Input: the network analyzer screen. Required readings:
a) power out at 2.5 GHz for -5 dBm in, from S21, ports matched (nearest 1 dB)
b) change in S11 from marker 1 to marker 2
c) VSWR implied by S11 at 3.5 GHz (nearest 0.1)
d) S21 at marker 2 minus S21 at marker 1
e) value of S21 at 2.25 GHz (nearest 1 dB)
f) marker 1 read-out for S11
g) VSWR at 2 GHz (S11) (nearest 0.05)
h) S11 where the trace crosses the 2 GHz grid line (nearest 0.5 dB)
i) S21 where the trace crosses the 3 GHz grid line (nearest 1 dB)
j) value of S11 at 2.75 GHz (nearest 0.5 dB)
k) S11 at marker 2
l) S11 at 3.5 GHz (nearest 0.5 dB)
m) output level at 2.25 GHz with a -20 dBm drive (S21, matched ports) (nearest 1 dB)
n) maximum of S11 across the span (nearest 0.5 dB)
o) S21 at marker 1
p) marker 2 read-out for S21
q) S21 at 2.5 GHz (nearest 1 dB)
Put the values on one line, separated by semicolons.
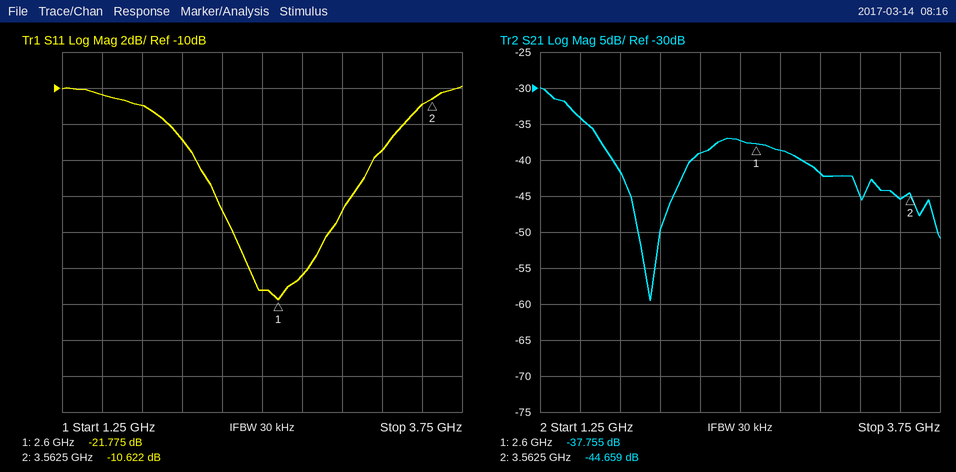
-42 dBm; 11.153 dB; 1.8; -6.904 dB; -39 dB; -21.775 dB; 1.60; -13.0 dB; -42 dB; -20.5 dB; -10.622 dB; -11.0 dB; -59 dBm; -10.0 dB; -37.755 dB; -44.659 dB; -37 dB
